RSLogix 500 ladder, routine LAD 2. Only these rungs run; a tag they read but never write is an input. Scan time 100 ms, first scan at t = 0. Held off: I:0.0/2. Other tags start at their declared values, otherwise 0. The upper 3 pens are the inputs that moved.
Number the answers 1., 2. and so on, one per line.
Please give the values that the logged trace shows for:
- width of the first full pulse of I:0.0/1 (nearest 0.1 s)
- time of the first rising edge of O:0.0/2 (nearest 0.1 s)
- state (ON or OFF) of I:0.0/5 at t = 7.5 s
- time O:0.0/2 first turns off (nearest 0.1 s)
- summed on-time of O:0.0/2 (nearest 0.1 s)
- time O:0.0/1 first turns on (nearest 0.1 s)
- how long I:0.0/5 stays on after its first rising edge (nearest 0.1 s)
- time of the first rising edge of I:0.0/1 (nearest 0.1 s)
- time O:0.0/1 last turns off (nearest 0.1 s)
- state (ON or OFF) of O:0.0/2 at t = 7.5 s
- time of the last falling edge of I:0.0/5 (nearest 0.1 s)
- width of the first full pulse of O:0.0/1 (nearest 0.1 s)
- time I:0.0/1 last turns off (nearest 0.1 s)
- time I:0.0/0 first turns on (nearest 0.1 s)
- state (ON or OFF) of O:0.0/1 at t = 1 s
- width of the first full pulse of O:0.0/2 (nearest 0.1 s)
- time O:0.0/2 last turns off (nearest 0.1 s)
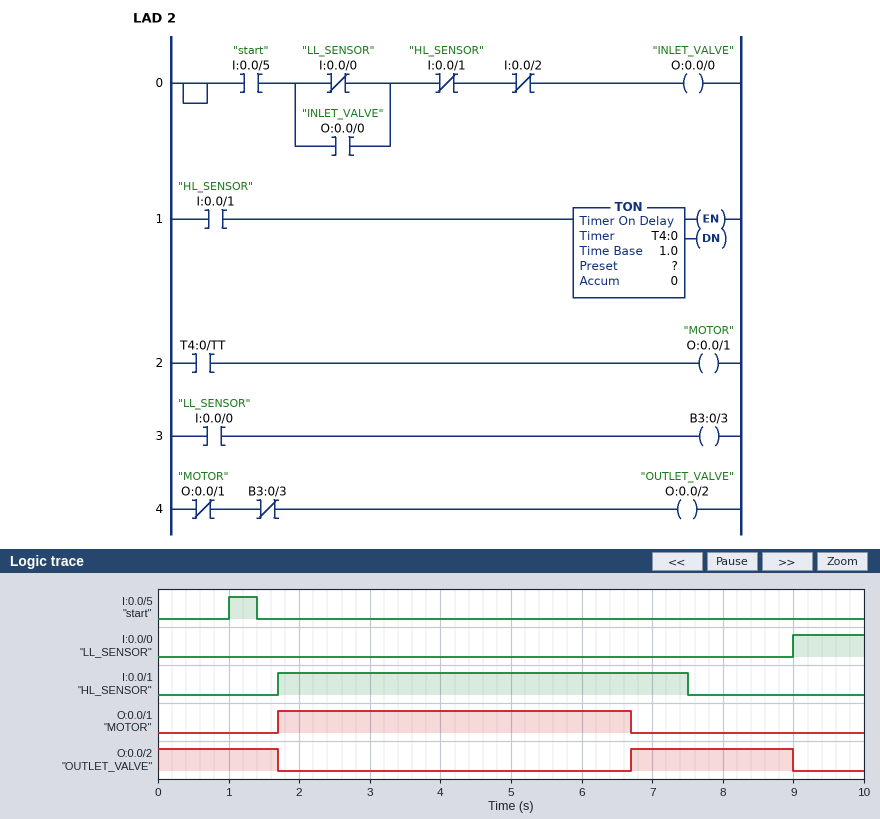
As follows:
1. 5.8 s
2. 6.7 s
3. OFF
4. 1.7 s
5. 4.0 s
6. 1.7 s
7. 0.4 s
8. 1.7 s
9. 6.7 s
10. ON
11. 1.4 s
12. 5.0 s
13. 7.5 s
14. 9.0 s
15. OFF
16. 2.3 s
17. 9.0 s
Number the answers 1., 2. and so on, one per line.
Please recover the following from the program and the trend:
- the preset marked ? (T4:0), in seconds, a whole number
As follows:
1. 5 s
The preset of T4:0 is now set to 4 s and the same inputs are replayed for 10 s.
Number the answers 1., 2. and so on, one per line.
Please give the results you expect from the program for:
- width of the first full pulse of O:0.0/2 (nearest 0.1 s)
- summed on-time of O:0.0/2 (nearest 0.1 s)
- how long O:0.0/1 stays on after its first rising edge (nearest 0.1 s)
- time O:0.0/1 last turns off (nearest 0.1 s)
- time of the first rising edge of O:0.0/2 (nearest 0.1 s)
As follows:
1. 3.3 s
2. 5.0 s
3. 4.0 s
4. 5.7 s
5. 5.7 s
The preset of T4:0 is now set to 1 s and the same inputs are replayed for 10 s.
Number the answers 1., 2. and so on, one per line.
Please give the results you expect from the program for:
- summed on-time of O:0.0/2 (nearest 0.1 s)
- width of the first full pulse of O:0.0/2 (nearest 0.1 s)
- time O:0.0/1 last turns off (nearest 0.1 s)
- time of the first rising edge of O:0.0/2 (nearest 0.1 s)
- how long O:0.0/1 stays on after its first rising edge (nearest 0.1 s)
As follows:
1. 8.0 s
2. 6.3 s
3. 2.7 s
4. 2.7 s
5. 1.0 s
